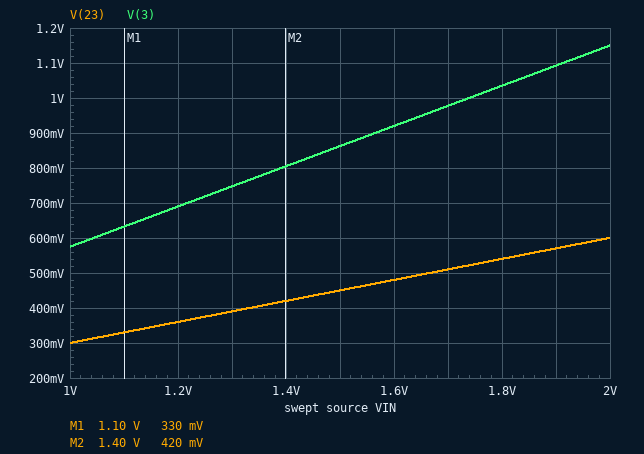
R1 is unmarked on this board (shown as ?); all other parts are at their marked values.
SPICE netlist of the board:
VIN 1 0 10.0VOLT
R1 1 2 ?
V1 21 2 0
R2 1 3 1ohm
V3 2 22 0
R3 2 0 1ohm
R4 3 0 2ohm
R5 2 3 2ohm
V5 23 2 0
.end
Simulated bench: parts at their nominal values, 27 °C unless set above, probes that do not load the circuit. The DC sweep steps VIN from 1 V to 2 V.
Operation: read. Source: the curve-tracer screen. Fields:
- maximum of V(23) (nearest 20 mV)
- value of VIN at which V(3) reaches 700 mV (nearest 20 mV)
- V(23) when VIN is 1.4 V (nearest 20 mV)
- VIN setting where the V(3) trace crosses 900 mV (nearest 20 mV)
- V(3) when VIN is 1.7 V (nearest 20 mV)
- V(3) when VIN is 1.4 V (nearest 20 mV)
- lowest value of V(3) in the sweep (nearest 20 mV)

600 mV
1.22 V
420 mV
1.56 V
980 mV
800 mV
580 mV
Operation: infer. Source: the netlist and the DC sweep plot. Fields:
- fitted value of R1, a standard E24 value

4.3 Ω
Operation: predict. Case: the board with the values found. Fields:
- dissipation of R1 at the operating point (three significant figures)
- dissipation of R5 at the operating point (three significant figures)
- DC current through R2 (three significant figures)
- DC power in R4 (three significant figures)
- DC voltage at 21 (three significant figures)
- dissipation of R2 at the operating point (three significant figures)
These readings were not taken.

11.4 W
3.78 W
4.25 A
16.5 W
3.00 V
18.1 W
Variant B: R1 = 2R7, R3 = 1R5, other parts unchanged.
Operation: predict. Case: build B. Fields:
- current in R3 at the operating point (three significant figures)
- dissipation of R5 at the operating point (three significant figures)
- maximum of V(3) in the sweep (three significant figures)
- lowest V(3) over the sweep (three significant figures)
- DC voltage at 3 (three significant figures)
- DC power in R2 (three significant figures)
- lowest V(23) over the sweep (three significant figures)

2.93 A
1.45 W
1.22 V
610 mV
6.10 V
15.2 W
439 mV
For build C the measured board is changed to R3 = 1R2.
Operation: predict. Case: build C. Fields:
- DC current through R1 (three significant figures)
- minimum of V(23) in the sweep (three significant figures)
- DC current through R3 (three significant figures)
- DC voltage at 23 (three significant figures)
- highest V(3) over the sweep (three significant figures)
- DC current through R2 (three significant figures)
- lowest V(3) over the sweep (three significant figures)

1.55 A
335 mV
2.79 A
3.35 V
1.17 V
4.16 A
584 mV
